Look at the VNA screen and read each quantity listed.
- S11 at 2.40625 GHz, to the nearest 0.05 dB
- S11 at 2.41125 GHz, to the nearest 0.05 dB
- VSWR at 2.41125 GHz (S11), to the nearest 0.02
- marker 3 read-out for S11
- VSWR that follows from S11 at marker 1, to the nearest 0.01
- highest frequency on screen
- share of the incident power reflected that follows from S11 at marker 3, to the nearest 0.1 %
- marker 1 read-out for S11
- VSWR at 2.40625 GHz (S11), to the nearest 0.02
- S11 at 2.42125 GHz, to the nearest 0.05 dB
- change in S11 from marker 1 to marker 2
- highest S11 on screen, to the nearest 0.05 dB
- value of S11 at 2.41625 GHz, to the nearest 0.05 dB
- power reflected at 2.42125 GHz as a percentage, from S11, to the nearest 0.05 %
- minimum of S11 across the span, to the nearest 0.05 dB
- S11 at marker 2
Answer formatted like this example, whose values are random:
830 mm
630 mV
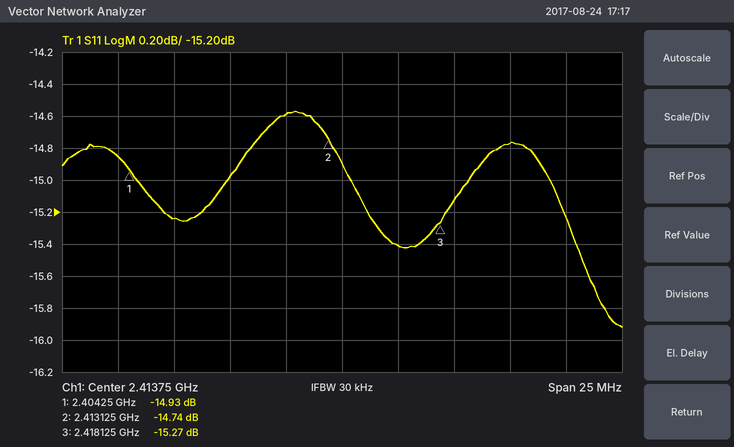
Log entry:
-15.25 dB
-14.60 dB
1.46
-15.27 dB
1.44
2.42625 GHz
3.0 %
-14.93 dB
1.42
-14.75 dB
0.19 dB
-14.55 dB
-15.40 dB
3.35 %
-15.90 dB
-14.74 dB
